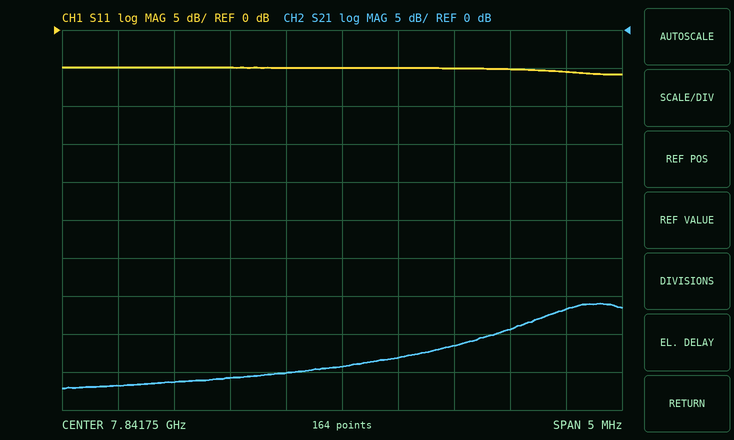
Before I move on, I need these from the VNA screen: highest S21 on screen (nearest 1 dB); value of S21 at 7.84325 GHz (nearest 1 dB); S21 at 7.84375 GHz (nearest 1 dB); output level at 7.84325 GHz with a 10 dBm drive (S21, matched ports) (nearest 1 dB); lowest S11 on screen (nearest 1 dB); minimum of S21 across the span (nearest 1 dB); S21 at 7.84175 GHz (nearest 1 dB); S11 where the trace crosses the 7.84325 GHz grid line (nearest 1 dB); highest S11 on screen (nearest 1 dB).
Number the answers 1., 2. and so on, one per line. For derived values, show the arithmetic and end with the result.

1. -36 dB
2. -39 dB
3. -37 dB
4. 10 dBm + (-39 dB) = -29 dBm
5. -6 dB
6. -47 dB
7. -44 dB
8. -5 dB
9. -5 dB
